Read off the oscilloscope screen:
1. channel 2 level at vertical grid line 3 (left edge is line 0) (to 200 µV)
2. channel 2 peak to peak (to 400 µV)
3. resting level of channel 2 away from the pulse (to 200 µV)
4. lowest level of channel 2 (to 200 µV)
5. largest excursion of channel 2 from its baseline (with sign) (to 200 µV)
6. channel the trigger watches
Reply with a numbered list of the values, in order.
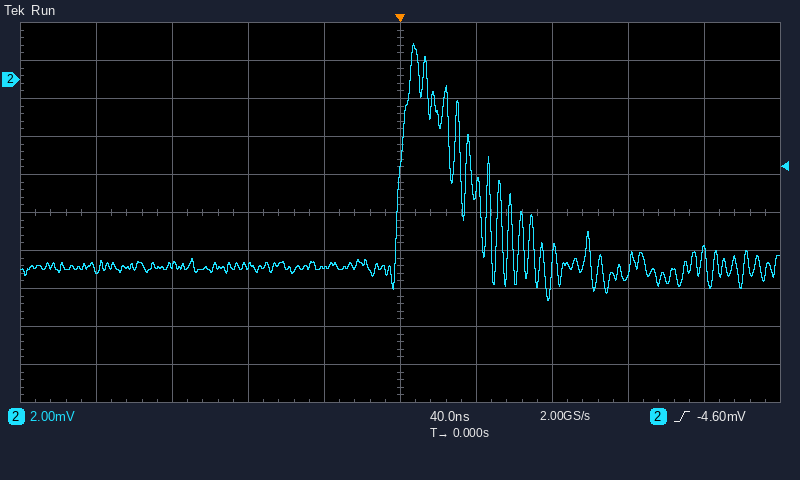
1. -9.8 mV
2. 13.6 mV
3. -9.8 mV
4. -11.6 mV
5. +11.8 mV
6. channel 2
